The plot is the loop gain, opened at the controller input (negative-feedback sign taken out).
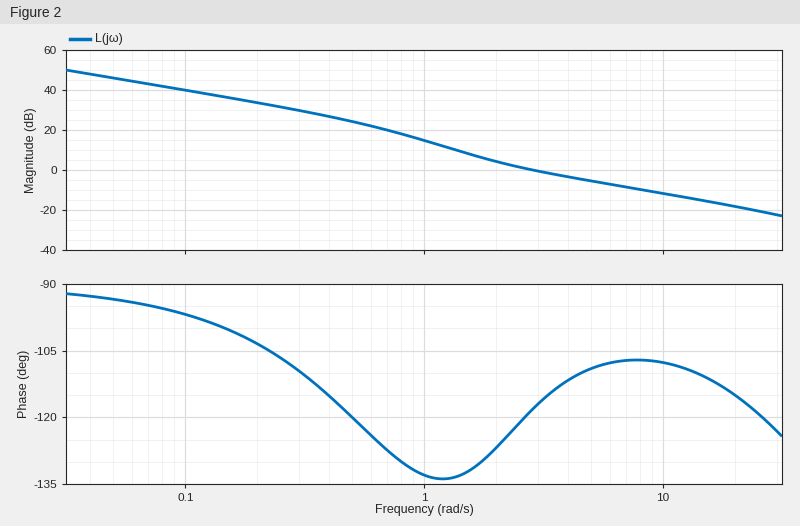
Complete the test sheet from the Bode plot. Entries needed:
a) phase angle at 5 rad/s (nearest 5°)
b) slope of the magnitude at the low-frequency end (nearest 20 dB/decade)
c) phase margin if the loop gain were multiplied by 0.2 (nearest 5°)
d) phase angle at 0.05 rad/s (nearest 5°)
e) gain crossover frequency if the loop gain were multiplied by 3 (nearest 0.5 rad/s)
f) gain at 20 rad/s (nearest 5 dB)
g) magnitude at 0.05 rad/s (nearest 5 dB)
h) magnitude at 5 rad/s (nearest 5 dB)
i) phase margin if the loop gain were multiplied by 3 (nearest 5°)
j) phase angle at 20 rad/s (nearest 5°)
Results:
-110°
-20 dB/decade
45°
-95°
8.0 rad/s
-20 dB
45 dB
-5 dB
75°
-115°
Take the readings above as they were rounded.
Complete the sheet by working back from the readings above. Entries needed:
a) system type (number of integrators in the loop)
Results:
1
